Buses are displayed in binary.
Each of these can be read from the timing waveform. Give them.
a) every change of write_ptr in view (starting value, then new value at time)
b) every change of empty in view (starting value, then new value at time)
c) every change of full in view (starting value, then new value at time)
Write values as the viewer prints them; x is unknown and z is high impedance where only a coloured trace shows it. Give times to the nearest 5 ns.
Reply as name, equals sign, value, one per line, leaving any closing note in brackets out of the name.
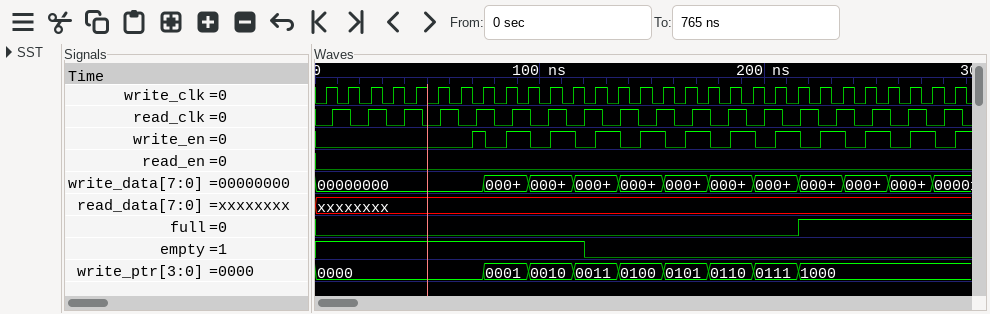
every change of write_ptr in view = 0000, 0001 at 75 ns, 0010 at 95 ns, 0011 at 115 ns, 0100 at 135 ns, 0101 at 155 ns, 0110 at 175 ns, 0111 at 195 ns, 1000 at 215 ns
every change of empty in view = 1, 0 at 120 ns
every change of full in view = 0, 1 at 215 ns
